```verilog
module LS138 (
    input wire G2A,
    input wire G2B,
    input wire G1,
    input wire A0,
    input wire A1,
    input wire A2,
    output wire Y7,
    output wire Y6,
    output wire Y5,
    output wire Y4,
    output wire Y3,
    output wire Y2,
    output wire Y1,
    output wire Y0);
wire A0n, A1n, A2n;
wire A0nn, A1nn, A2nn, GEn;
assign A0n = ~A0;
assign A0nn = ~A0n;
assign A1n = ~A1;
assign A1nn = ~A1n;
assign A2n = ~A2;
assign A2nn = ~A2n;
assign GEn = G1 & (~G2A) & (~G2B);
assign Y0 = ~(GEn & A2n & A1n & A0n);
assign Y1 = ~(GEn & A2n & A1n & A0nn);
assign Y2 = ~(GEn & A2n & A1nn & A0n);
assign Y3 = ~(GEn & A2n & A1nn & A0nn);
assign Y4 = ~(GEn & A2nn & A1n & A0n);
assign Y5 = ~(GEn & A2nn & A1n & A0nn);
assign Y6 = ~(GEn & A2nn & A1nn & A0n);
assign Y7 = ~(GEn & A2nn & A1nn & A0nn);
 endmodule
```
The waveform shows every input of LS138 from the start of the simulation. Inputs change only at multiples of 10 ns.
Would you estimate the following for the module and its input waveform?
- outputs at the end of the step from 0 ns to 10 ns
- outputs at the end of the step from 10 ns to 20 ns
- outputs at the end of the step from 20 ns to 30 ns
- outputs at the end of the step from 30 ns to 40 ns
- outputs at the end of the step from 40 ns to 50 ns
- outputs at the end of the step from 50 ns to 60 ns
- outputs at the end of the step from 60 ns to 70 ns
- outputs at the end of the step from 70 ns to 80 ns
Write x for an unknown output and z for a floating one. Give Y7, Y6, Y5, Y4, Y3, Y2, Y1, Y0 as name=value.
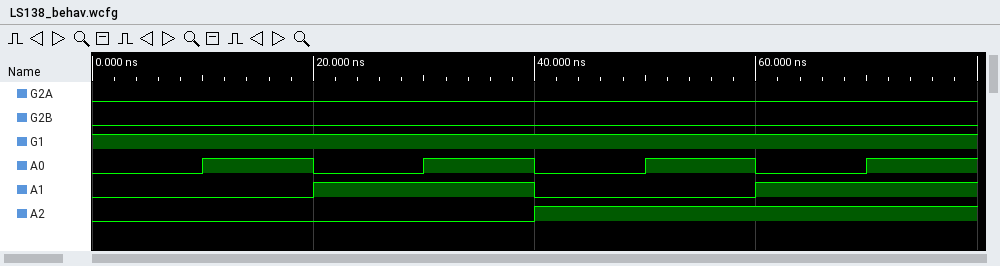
Y7=1, Y6=1, Y5=1, Y4=1, Y3=1, Y2=1, Y1=1, Y0=0
Y7=1, Y6=1, Y5=1, Y4=1, Y3=1, Y2=1, Y1=0, Y0=1
Y7=1, Y6=1, Y5=1, Y4=1, Y3=1, Y2=0, Y1=1, Y0=1
Y7=1, Y6=1, Y5=1, Y4=1, Y3=0, Y2=1, Y1=1, Y0=1
Y7=1, Y6=1, Y5=1, Y4=0, Y3=1, Y2=1, Y1=1, Y0=1
Y7=1, Y6=1, Y5=0, Y4=1, Y3=1, Y2=1, Y1=1, Y0=1
Y7=1, Y6=0, Y5=1, Y4=1, Y3=1, Y2=1, Y1=1, Y0=1
Y7=0, Y6=1, Y5=1, Y4=1, Y3=1, Y2=1, Y1=1, Y0=1
